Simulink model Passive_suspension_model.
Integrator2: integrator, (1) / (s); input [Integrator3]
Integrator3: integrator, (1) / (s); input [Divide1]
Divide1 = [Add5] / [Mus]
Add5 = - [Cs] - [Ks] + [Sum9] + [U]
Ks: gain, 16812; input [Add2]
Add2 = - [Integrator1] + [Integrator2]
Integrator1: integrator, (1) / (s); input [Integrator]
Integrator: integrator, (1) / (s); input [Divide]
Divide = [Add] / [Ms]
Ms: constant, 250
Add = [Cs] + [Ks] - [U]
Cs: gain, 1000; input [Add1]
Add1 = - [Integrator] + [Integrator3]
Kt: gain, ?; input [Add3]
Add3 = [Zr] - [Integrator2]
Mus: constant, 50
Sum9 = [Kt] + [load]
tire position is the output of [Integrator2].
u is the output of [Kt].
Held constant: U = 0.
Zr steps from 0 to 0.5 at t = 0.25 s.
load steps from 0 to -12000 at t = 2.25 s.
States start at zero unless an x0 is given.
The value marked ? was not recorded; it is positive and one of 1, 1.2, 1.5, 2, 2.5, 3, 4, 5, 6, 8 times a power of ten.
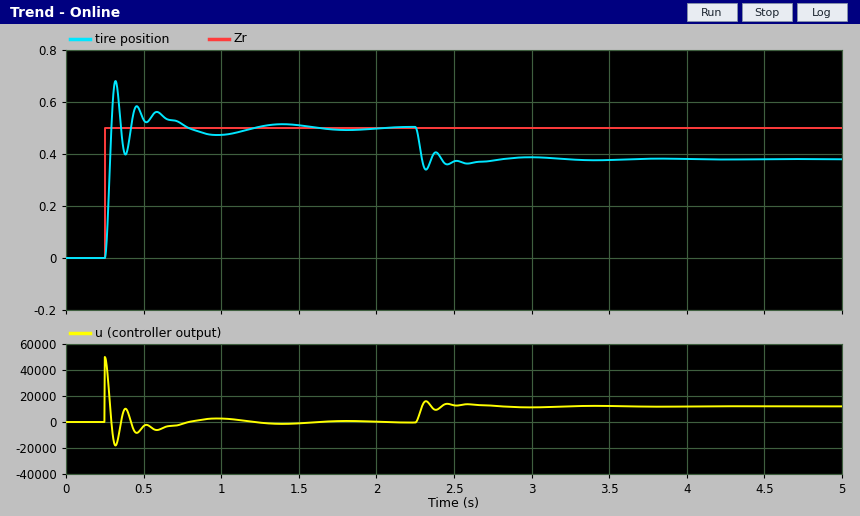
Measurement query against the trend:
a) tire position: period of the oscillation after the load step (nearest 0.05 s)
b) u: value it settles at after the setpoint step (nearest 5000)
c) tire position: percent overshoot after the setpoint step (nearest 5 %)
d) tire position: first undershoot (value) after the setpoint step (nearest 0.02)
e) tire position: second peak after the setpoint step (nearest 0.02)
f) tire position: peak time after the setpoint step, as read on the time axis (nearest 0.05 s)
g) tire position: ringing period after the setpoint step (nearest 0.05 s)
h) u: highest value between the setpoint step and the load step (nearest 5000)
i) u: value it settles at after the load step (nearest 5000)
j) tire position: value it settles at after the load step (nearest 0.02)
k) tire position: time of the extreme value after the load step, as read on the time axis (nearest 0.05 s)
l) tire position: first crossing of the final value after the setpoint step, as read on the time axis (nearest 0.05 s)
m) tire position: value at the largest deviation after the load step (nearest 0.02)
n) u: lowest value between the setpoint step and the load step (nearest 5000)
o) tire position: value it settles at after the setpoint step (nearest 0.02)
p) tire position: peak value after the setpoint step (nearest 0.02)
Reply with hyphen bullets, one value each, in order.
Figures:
- 0.15 s
- 0
- 35 %
- 0.40
- 0.58
- 0.30 s
- 0.15 s
- 50000
- 10000
- 0.38
- 2.30 s
- 0.30 s
- 0.34
- -20000
- 0.50
- 0.68
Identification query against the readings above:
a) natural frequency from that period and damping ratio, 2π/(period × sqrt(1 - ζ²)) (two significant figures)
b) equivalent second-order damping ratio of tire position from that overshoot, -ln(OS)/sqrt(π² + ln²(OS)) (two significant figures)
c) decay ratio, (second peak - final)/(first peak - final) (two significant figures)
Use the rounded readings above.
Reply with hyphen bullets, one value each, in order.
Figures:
- 44 rad/s
- 0.32
- 0.44
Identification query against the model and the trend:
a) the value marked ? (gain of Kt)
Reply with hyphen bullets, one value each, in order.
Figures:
- 100000
